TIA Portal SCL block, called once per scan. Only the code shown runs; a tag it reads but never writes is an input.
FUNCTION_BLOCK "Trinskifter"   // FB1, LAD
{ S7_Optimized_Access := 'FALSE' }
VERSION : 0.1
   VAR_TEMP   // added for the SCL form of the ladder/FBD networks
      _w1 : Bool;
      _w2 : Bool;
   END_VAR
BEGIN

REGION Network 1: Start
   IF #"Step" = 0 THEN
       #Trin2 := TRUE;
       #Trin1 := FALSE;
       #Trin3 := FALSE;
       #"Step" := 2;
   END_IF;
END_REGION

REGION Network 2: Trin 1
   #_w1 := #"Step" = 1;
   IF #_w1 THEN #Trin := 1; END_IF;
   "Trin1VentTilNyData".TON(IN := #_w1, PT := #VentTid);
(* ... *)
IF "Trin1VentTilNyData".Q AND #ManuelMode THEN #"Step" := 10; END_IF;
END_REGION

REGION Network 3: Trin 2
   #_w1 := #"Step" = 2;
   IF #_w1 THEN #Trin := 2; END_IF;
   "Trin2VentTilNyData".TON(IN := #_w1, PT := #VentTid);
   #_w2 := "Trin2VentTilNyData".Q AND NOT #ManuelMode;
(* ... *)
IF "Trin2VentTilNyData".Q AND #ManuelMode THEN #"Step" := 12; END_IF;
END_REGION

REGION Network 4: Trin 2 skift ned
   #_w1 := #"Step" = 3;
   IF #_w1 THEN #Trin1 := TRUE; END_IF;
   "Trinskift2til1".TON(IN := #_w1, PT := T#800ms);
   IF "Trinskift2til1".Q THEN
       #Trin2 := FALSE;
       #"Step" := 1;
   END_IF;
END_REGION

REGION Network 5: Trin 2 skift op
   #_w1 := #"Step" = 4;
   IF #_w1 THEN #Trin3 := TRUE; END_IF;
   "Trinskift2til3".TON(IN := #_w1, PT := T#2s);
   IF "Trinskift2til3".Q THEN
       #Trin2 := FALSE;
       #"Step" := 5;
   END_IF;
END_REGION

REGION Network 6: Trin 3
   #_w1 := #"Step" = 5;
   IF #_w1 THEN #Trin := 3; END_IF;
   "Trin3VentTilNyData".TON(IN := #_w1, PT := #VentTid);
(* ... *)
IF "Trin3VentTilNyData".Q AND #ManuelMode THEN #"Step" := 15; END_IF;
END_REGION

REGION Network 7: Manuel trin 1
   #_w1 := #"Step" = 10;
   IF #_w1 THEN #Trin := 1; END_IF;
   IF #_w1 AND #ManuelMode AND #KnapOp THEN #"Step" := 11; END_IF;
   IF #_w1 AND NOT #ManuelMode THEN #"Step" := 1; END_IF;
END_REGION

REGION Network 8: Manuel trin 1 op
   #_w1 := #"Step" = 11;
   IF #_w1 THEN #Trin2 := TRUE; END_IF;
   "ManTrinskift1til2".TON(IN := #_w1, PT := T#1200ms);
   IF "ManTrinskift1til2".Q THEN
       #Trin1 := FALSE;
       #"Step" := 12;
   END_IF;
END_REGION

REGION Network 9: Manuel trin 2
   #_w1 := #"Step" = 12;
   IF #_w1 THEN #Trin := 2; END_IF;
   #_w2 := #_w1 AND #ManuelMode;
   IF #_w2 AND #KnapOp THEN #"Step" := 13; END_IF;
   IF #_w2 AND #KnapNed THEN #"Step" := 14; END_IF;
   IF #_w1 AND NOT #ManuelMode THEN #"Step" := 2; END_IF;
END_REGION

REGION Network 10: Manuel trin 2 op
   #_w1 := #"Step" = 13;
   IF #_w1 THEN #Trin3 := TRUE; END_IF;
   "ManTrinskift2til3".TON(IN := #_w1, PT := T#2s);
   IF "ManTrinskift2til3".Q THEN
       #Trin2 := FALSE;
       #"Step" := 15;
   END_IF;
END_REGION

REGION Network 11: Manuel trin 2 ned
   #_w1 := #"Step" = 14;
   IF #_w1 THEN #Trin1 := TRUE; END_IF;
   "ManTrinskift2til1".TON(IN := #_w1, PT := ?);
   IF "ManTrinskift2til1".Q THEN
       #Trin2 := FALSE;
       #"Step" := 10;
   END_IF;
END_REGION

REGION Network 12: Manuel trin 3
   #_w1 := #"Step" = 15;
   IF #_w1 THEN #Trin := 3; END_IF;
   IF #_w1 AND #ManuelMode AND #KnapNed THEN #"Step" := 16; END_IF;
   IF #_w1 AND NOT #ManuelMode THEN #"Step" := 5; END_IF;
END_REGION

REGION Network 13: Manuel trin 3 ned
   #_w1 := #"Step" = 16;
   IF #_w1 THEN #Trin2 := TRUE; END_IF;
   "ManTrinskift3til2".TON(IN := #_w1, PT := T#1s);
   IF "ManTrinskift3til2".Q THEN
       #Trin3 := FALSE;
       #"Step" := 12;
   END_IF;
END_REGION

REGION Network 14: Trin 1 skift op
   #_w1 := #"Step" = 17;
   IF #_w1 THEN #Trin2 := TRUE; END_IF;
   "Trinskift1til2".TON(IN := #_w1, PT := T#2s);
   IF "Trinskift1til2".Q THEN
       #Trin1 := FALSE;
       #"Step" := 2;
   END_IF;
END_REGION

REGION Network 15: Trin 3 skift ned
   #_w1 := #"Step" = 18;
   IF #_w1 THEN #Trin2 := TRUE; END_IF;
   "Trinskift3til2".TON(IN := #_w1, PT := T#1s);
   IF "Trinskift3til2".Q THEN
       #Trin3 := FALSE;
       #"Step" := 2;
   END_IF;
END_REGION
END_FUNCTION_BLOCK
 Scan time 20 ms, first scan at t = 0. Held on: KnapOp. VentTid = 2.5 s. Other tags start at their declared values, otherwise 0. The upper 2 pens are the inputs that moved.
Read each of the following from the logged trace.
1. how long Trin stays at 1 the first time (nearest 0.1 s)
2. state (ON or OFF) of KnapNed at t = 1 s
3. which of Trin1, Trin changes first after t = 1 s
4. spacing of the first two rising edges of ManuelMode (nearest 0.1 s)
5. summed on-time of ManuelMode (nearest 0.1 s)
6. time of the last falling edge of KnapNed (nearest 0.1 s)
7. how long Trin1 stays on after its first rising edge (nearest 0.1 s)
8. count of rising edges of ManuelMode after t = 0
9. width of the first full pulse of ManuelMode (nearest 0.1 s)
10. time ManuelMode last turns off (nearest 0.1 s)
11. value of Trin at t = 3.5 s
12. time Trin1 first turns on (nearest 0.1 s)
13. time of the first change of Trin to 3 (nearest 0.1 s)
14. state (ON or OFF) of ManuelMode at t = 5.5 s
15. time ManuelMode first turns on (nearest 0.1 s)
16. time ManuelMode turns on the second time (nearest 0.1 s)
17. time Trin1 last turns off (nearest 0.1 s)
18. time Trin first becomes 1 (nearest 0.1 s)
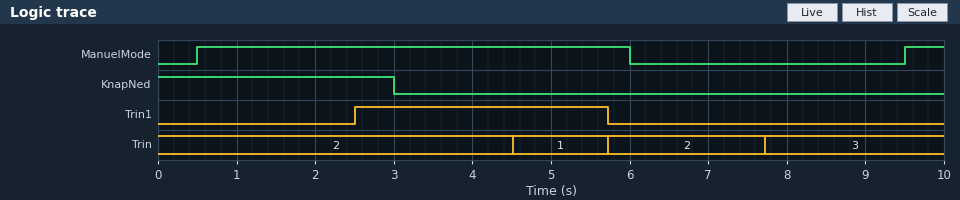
1.2 s
ON
Trin1
9.0 s
6.0 s
3.0 s
3.2 s
2
5.5 s
6.0 s
2
2.5 s
7.7 s
ON
0.5 s
9.5 s
5.7 s
4.5 s
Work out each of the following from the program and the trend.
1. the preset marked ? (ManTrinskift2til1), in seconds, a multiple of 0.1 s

2.0 s
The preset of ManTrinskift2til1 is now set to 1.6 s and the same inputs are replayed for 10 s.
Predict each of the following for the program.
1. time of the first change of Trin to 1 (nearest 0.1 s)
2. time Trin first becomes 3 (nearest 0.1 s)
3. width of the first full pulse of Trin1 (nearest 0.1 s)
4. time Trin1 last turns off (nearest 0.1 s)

4.1 s
7.3 s
2.8 s
5.3 s
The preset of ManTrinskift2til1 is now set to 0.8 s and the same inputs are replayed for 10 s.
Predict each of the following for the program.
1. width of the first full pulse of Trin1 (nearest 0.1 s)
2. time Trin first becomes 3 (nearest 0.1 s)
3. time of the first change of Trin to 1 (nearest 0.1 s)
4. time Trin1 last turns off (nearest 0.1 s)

2.0 s
6.5 s
3.3 s
4.5 s
